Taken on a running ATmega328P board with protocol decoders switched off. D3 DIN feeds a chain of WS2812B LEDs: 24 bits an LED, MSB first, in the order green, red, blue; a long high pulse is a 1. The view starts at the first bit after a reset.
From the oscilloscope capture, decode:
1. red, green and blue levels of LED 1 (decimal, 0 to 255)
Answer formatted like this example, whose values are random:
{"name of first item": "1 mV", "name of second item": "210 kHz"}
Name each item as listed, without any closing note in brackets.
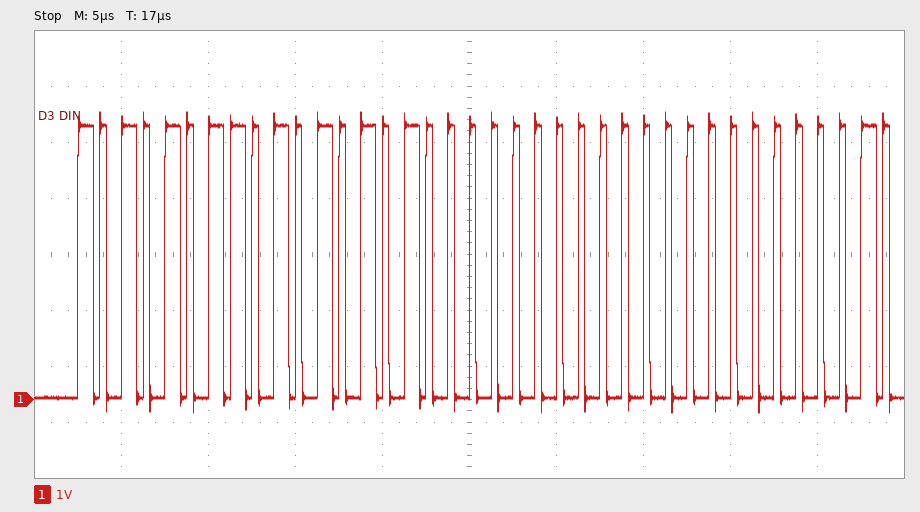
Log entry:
{"red, green and blue levels of LED 1": "85, 171, 0"}
